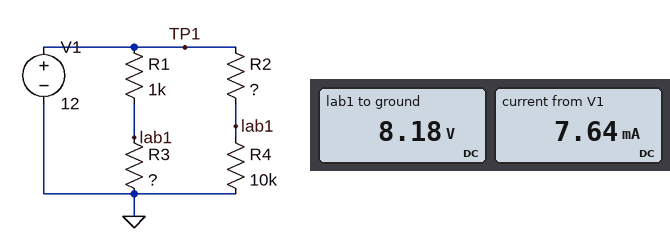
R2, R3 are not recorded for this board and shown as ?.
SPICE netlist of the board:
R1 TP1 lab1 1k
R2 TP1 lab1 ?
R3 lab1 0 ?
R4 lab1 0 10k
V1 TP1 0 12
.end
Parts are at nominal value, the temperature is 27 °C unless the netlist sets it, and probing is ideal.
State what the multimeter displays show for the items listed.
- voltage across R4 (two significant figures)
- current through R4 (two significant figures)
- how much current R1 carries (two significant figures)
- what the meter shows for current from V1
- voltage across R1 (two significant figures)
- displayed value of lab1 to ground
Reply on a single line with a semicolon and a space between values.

8.2 V; 820 µA; 3.8 mA; 7.64 mA; 3.8 V; 8.18 V
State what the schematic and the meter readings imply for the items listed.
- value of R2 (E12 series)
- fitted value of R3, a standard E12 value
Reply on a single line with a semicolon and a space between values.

1 kΩ; 1.2 kΩ
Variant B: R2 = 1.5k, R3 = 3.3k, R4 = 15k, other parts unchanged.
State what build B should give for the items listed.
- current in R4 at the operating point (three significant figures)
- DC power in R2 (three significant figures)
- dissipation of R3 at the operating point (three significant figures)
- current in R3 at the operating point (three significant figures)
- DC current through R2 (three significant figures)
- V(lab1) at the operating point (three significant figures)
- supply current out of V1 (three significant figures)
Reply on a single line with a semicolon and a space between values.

655 µA; 3.16 mW; 29.2 mW; 2.98 mA; 1.45 mA; 9.82 V; 3.63 mA
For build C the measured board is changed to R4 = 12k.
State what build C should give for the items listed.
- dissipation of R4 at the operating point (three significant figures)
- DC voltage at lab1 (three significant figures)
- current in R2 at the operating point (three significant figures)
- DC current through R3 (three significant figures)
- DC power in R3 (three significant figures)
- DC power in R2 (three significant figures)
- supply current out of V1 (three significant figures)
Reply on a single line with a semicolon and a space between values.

5.64 mW; 8.23 V; 3.77 mA; 6.86 mA; 56.4 mW; 14.2 mW; 7.54 mA
